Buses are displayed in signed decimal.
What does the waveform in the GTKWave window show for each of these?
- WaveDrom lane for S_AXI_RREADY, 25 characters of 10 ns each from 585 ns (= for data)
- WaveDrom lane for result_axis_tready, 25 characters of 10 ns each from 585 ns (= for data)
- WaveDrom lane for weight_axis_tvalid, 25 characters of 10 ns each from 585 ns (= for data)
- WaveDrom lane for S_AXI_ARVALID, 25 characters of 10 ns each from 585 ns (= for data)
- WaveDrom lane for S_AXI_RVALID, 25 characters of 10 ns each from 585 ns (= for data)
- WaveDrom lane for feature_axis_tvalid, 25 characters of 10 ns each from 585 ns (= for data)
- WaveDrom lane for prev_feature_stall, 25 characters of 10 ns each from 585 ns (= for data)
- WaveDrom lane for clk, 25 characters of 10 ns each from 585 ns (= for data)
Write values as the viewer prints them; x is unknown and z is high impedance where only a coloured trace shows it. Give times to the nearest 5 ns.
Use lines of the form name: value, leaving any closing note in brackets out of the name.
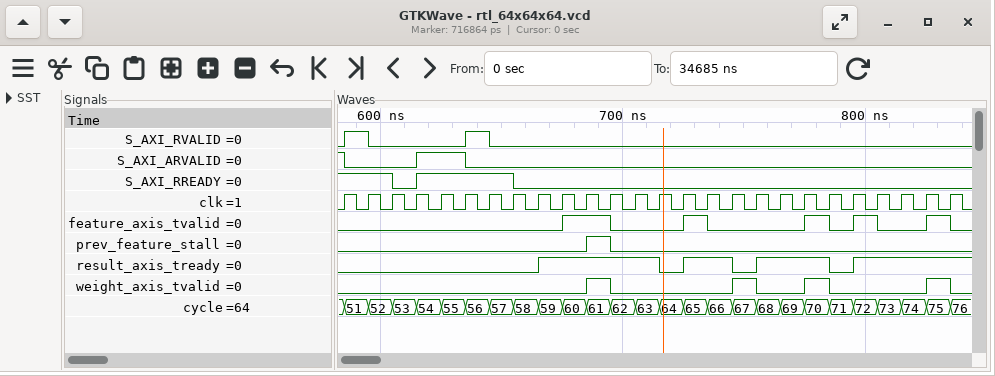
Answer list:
WaveDrom lane for S_AXI_RREADY, 25 characters of 10 ns each from 585 ns: {name: 'S_AXI_RREADY', wave: '1.01...0.................'}
WaveDrom lane for result_axis_tready, 25 characters of 10 ns each from 585 ns: {name: 'result_axis_tready', wave: '0.......1....01.01..01...'}
WaveDrom lane for weight_axis_tvalid, 25 characters of 10 ns each from 585 ns: {name: 'weight_axis_tvalid', wave: '0.........10....10.10...1'}
WaveDrom lane for S_AXI_ARVALID, 25 characters of 10 ns each from 585 ns: {name: 'S_AXI_ARVALID', wave: '0..1.0...................'}
WaveDrom lane for S_AXI_RVALID, 25 characters of 10 ns each from 585 ns: {name: 'S_AXI_RVALID', wave: '10...10..................'}
WaveDrom lane for feature_axis_tvalid, 25 characters of 10 ns each from 585 ns: {name: 'feature_axis_tvalid', wave: '0........1.0..10...1010.1'}
WaveDrom lane for prev_feature_stall, 25 characters of 10 ns each from 585 ns: {name: 'prev_feature_stall', wave: '0.........10.............'}
WaveDrom lane for clk, 25 characters of 10 ns each from 585 ns: {name: 'clk', wave: 'p........................'}
